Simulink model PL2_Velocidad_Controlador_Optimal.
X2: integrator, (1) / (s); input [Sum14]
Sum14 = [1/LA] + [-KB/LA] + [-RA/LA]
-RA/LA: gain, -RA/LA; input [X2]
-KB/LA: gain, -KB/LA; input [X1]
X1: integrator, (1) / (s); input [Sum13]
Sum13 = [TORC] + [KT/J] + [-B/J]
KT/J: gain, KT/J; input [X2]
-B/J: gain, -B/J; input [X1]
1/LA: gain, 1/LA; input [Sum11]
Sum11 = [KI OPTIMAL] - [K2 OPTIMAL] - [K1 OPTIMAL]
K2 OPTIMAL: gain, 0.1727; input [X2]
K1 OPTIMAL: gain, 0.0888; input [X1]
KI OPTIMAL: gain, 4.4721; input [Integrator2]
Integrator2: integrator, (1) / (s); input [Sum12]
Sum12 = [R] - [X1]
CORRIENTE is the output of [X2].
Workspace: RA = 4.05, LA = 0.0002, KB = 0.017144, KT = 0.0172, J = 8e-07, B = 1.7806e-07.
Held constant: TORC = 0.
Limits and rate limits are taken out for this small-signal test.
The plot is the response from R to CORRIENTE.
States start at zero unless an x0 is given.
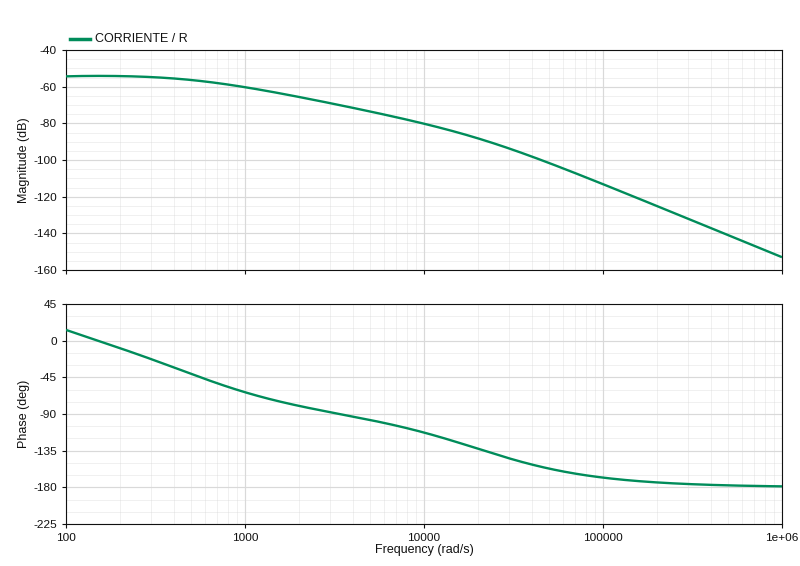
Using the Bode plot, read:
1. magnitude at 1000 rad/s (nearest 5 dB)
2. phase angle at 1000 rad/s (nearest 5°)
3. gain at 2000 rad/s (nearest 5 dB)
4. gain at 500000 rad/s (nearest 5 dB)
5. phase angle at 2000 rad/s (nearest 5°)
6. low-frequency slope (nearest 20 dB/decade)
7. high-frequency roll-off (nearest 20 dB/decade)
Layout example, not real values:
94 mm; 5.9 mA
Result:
-60 dB; -65°; -65 dB; -140 dB; -80°; 0 dB/decade; -40 dB/decade
